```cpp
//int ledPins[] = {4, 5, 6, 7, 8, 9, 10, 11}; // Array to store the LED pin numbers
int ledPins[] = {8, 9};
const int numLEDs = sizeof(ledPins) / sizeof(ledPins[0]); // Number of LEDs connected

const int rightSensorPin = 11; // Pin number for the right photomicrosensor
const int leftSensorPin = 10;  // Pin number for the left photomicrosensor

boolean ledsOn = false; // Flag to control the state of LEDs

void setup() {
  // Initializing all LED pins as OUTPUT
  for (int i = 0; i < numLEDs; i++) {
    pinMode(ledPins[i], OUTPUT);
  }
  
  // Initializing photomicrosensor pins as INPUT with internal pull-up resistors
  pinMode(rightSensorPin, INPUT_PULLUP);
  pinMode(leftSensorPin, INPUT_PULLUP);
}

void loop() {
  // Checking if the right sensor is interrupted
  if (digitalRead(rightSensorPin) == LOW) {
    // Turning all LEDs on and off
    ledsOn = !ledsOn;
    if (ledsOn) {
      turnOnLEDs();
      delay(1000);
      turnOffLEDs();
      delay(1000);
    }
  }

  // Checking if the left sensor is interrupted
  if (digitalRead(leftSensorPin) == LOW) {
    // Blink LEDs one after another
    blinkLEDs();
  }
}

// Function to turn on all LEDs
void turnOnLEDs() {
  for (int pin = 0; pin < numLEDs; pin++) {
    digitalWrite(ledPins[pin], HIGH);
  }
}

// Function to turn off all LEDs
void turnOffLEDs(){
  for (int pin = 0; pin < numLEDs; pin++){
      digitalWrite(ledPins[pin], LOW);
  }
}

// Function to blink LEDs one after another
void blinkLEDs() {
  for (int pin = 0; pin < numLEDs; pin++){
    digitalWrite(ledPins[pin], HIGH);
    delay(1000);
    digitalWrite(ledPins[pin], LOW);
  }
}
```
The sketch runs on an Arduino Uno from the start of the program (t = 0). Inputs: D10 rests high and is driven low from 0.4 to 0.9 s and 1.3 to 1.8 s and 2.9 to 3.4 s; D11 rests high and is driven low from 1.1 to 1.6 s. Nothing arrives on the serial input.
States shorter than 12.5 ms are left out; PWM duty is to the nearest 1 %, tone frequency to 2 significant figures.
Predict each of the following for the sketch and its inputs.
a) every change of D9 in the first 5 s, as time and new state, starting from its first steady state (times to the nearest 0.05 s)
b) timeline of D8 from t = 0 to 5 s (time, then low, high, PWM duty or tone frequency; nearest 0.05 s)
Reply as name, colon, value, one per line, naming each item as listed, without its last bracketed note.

every change of D9 in the first 5 s, as time and new state, starting from its first steady state: 0 s low; 1.4 s high; 2.4 s low; 3.9 s high; 4.9 s low
timeline of D8 from t = 0 to 5 s: 0 s low; 0.4 s high; 1.4 s low; 2.9 s high; 3.9 s low
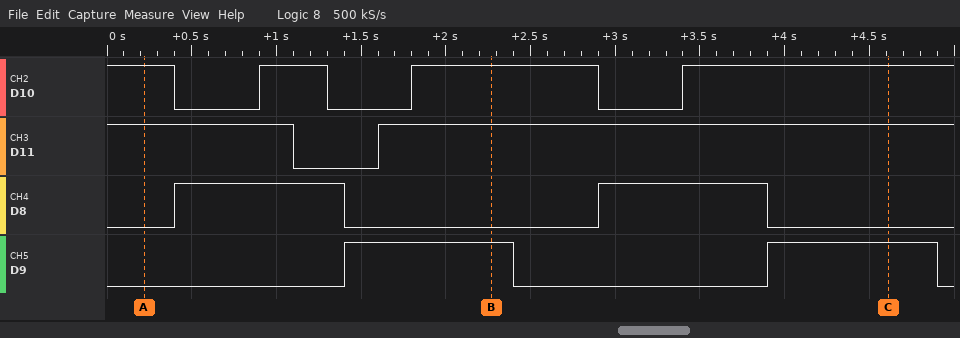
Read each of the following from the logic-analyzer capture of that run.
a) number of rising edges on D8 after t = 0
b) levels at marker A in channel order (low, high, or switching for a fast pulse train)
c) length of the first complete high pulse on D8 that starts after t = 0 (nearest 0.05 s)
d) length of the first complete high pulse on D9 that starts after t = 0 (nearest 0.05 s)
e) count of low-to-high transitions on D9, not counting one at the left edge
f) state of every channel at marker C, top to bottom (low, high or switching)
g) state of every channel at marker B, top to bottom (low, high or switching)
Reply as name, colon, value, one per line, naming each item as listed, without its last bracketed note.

number of rising edges on D8 after t = 0: 2
levels at marker A in channel order: D10 high, D11 high, D8 low, D9 low
length of the first complete high pulse on D8 that starts after t = 0: 1.00 s
length of the first complete high pulse on D9 that starts after t = 0: 1.00 s
count of low-to-high transitions on D9, not counting one at the left edge: 2
state of every channel at marker C, top to bottom: D10 high, D11 high, D8 low, D9 high
state of every channel at marker B, top to bottom: D10 high, D11 high, D8 low, D9 high
